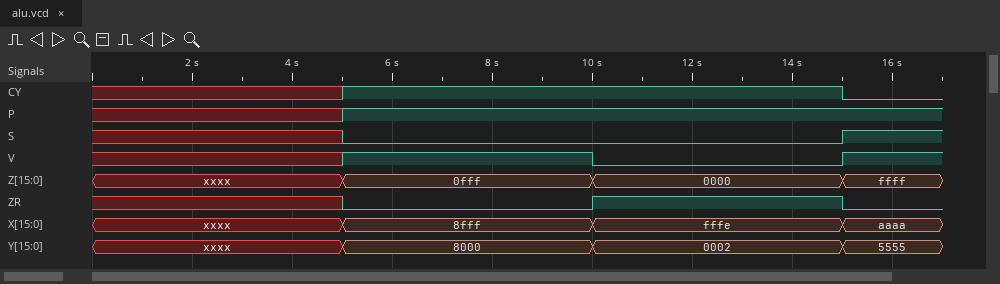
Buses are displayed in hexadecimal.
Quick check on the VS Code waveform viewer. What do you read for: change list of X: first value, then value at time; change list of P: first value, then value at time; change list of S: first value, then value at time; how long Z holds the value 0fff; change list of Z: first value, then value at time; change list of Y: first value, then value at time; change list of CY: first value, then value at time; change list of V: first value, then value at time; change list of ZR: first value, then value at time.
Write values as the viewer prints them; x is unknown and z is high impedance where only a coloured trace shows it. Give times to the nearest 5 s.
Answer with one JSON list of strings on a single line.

["xxxx, 8fff at 5 s, fffe at 10 s, aaaa at 15 s", "x, 1 at 5 s", "x, 0 at 5 s, 1 at 15 s", "5 s", "xxxx, 0fff at 5 s, 0000 at 10 s, ffff at 15 s", "xxxx, 8000 at 5 s, 0002 at 10 s, 5555 at 15 s", "x, 1 at 5 s, 0 at 15 s", "x, 1 at 5 s, 0 at 10 s, 1 at 15 s", "x, 0 at 5 s, 1 at 10 s, 0 at 15 s"]
